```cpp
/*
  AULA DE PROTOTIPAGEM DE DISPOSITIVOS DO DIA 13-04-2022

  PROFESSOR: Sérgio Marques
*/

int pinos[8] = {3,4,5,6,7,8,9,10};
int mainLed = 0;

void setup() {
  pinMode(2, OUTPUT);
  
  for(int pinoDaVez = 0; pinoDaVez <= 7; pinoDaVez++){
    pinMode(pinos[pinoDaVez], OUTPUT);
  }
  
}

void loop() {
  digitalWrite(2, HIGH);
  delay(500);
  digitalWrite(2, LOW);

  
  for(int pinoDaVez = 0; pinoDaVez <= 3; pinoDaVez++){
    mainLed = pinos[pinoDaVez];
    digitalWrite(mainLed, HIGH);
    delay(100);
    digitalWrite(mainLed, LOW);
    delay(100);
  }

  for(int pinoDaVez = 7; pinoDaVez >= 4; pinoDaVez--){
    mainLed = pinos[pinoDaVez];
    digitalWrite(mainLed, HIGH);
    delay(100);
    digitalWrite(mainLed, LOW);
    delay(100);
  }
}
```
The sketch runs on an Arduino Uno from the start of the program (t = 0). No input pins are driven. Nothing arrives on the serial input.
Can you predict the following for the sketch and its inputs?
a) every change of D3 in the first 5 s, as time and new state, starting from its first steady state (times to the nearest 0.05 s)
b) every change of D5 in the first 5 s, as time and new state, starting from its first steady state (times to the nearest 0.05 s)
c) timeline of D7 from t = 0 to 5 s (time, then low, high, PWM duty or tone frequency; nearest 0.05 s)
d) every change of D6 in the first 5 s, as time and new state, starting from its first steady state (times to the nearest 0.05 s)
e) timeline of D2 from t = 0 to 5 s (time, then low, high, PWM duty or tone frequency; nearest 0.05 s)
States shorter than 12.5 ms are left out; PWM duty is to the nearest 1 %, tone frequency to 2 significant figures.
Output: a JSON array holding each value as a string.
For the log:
["0 s low; 0.5 s high; 0.6 s low; 2.6 s high; 2.7 s low; 4.7 s high; 4.8 s low", "0 s low; 0.9 s high; 1 s low; 3 s high; 3.1 s low", "0 s low; 1.9 s high; 2 s low; 4 s high; 4.1 s low", "0 s low; 1.1 s high; 1.2 s low; 3.2 s high; 3.3 s low", "0 s high; 0.5 s low; 2.1 s high; 2.6 s low; 4.2 s high; 4.7 s low"]
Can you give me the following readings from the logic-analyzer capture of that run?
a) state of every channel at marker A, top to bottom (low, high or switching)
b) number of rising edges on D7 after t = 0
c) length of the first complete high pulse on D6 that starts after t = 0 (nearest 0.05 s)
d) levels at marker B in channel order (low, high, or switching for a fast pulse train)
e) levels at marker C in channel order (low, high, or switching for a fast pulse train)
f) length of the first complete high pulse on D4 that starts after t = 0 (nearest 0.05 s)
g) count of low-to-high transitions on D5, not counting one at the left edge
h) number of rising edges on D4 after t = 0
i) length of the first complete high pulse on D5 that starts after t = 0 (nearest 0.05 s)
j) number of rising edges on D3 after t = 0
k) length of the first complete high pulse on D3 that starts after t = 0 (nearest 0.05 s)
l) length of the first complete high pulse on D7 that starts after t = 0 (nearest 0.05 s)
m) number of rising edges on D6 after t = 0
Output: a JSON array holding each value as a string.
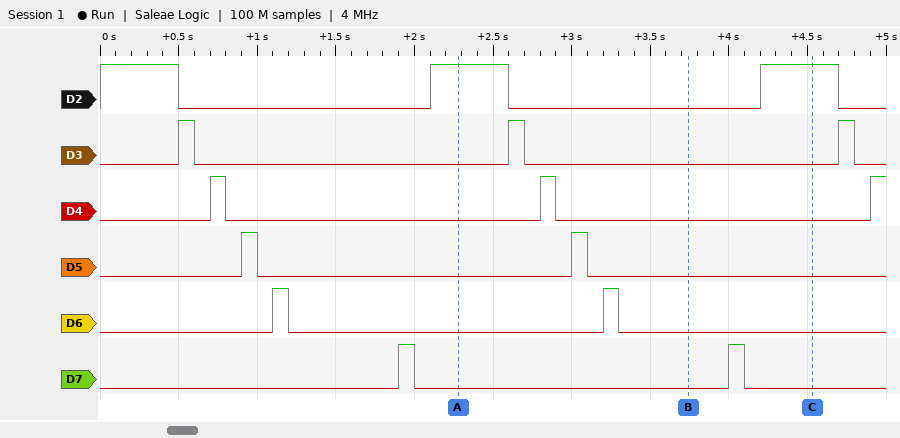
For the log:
["D2 high, D3 low, D4 low, D5 low, D6 low, D7 low", "2", "0.10 s", "D2 low, D3 low, D4 low, D5 low, D6 low, D7 low", "D2 high, D3 low, D4 low, D5 low, D6 low, D7 low", "0.10 s", "2", "3", "0.10 s", "3", "0.10 s", "0.10 s", "2"]
